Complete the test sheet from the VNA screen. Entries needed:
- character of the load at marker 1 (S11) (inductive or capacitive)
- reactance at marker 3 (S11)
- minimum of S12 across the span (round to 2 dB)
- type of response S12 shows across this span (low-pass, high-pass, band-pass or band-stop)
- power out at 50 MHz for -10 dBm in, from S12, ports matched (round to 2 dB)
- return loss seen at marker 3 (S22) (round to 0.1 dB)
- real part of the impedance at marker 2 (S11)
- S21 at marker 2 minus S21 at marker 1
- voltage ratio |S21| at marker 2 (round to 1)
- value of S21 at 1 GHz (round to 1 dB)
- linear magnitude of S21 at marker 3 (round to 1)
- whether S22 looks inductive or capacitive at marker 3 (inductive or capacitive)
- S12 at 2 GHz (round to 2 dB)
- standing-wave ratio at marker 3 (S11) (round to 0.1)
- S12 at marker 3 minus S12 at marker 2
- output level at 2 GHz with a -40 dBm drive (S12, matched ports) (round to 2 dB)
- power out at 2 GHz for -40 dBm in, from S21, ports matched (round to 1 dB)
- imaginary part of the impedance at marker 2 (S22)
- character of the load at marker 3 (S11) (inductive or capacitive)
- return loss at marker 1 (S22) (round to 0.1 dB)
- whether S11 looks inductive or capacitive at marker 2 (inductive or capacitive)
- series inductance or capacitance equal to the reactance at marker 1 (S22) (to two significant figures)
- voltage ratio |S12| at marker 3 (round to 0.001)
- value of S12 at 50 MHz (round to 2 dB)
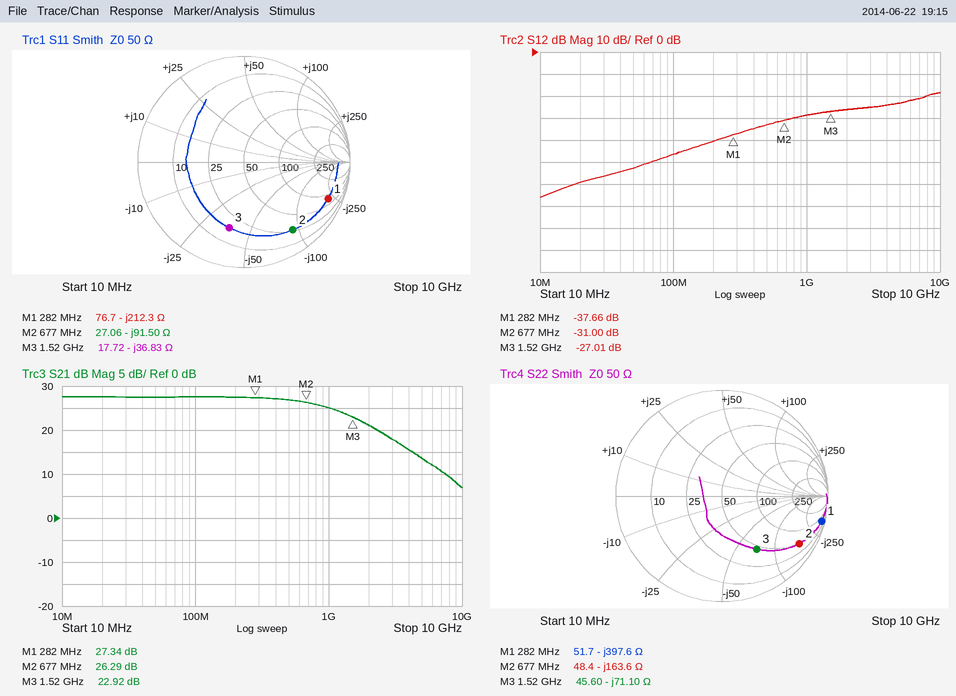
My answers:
capacitive
-36.83 Ω
-66 dB
high-pass
-62 dBm
4.5 dB
27.06 Ω
-1.05 dB
21
25 dB
14
capacitive
-26 dB
4.5
3.99 dB
-66 dBm
-19 dBm
-163.6 Ω
capacitive
0.3 dB
capacitive
1.4 pF
0.045
-52 dB
